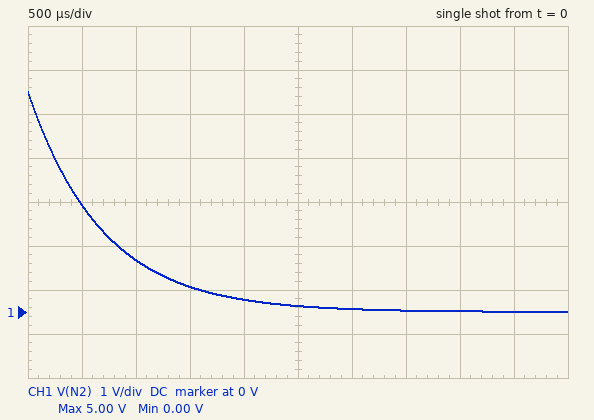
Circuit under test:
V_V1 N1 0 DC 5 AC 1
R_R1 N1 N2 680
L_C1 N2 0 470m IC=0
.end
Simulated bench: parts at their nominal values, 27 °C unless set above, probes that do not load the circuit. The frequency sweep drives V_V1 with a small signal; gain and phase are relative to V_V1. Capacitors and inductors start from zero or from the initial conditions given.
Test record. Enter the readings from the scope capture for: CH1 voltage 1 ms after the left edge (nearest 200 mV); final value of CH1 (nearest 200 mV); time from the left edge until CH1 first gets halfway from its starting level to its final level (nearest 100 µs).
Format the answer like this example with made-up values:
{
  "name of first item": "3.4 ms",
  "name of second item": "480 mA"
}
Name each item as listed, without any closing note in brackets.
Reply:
{
  "CH1 voltage 1 ms after the left edge": "1.2 V",
  "final value of CH1": "0 V",
  "time from the left edge until CH1 first gets halfway from its starting level to its final level": "500 µs"
}
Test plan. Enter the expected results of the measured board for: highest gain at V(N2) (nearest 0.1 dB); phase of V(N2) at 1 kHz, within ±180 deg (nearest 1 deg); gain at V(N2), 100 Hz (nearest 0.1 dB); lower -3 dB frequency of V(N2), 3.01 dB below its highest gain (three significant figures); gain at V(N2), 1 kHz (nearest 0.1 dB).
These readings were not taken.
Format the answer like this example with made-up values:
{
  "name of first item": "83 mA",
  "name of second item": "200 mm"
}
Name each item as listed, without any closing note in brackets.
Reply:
{
  "highest gain at V(N2)": "0 dB",
  "phase of V(N2) at 1 kHz, within ±180 deg": "13 deg",
  "gain at V(N2), 100 Hz": "-8.0 dB",
  "lower -3 dB frequency of V(N2), 3.01 dB below its highest gain": "230 Hz",
  "gain at V(N2), 1 kHz": "-0.2 dB"
}
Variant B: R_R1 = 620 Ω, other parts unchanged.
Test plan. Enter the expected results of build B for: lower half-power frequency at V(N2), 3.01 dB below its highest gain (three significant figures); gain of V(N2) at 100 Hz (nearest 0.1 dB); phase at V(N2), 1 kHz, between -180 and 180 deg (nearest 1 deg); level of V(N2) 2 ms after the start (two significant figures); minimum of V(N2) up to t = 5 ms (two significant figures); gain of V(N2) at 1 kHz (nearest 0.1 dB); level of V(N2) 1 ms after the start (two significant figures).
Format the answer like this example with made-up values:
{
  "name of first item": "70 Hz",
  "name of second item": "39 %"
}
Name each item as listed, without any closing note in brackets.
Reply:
{
  "lower half-power frequency at V(N2), 3.01 dB below its highest gain": "210 Hz",
  "gain of V(N2) at 100 Hz": "-7.3 dB",
  "phase at V(N2), 1 kHz, between -180 and 180 deg": "12 deg",
  "level of V(N2) 2 ms after the start": "360 mV",
  "minimum of V(N2) up to t = 5 ms": "6.8 mV",
  "gain of V(N2) at 1 kHz": "-0.2 dB",
  "level of V(N2) 1 ms after the start": "1.3 V"
}
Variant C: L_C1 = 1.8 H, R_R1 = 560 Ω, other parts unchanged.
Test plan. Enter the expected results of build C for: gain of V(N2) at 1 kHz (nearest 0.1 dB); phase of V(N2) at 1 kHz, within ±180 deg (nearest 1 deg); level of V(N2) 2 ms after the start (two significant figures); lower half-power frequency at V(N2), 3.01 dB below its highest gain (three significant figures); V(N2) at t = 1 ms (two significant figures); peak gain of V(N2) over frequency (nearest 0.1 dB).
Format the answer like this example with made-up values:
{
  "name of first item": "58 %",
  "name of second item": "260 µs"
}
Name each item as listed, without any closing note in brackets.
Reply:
{
  "gain of V(N2) at 1 kHz": "0 dB",
  "phase of V(N2) at 1 kHz, within ±180 deg": "3 deg",
  "level of V(N2) 2 ms after the start": "2.7 V",
  "lower half-power frequency at V(N2), 3.01 dB below its highest gain": "49.5 Hz",
  "V(N2) at t = 1 ms": "3.7 V",
  "peak gain of V(N2) over frequency": "0 dB"
}
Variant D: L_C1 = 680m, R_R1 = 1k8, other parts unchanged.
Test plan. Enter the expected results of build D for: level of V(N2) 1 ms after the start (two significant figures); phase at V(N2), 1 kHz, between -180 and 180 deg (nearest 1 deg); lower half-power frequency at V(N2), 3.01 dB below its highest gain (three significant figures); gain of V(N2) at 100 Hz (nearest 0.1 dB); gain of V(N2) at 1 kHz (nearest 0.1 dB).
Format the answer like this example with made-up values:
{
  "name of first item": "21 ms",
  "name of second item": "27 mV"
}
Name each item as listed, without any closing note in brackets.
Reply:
{
  "level of V(N2) 1 ms after the start": "350 mV",
  "phase at V(N2), 1 kHz, between -180 and 180 deg": "23 deg",
  "lower half-power frequency at V(N2), 3.01 dB below its highest gain": "421 Hz",
  "gain of V(N2) at 100 Hz": "-12.7 dB",
  "gain of V(N2) at 1 kHz": "-0.7 dB"
}
